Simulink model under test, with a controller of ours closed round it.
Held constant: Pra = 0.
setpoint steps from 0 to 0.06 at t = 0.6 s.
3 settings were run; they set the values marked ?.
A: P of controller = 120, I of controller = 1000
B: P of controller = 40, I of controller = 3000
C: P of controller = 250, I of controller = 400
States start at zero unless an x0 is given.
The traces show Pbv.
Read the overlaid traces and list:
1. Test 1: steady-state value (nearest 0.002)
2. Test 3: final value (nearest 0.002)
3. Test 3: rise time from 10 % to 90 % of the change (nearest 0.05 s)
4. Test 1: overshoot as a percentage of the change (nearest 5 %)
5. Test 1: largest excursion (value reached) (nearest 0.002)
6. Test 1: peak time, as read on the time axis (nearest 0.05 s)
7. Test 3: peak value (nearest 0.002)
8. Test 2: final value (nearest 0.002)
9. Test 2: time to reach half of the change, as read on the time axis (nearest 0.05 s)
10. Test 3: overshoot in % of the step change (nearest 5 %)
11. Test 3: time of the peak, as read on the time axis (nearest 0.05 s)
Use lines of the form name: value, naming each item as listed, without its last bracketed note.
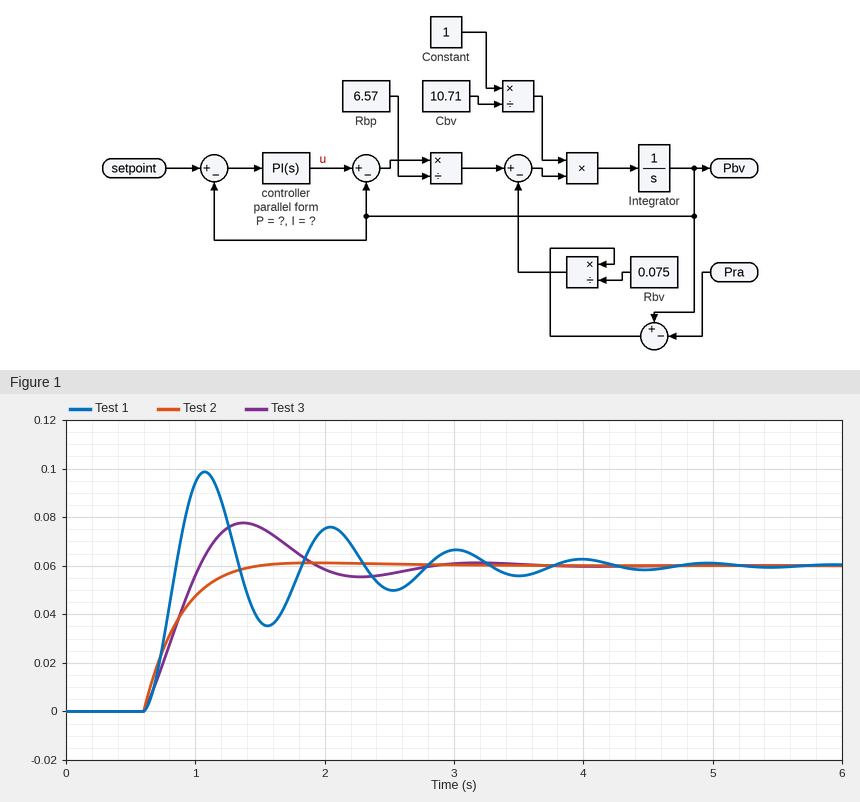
Test 1: steady-state value: 0.060
Test 3: final value: 0.060
Test 3: rise time from 10 % to 90 % of the change: 0.35 s
Test 1: overshoot as a percentage of the change: 65 %
Test 1: largest excursion (value reached): 0.098
Test 1: peak time, as read on the time axis: 1.05 s
Test 3: peak value: 0.078
Test 2: final value: 0.060
Test 2: time to reach half of the change, as read on the time axis: 0.80 s
Test 3: overshoot in % of the step change: 30 %
Test 3: time of the peak, as read on the time axis: 1.35 s
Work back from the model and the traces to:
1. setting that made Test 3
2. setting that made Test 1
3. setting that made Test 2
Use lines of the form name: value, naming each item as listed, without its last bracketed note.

setting that made Test 3: A
setting that made Test 1: B
setting that made Test 2: C
